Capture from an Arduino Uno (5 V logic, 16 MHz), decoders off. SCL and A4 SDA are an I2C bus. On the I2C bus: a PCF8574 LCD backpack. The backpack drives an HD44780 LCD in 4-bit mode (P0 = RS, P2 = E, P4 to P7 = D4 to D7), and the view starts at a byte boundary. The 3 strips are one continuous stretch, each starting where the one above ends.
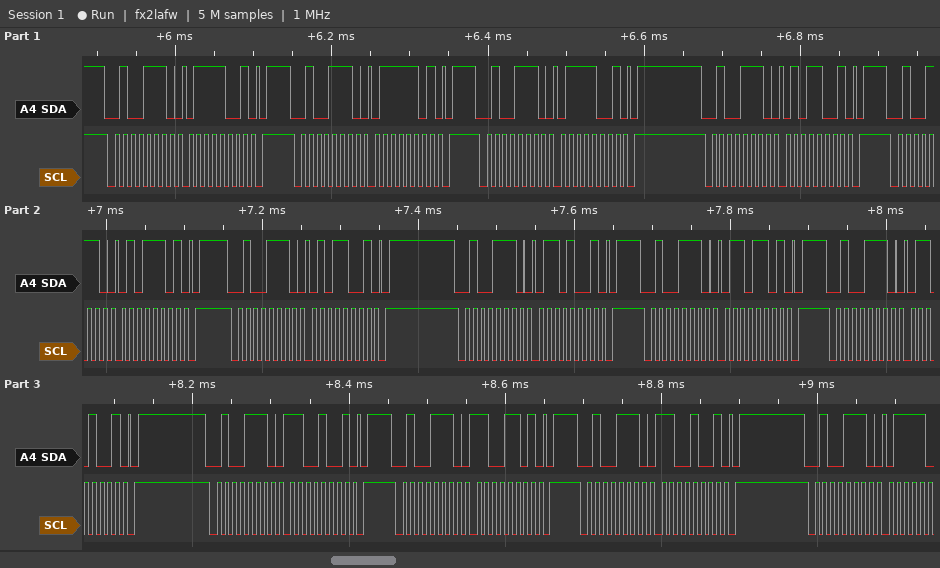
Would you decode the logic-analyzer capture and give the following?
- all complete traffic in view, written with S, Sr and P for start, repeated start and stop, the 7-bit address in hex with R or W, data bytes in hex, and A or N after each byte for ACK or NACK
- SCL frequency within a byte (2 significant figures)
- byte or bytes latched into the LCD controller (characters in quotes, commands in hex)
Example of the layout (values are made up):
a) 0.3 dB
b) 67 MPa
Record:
a) S 27W A 79 A P S 27W A 7D A P S 27W A 79 A P S 27W A 59 A P S 27W A 5D A P S 27W A 59 A P S 27W A 69 A P S 27W A 6D A P S 27W A 69 A P S 27W A C9 A P S 27W A CD A P S 27W A C9 A P S 27W A
b) 100 kHz
c) 'u' 'l'
